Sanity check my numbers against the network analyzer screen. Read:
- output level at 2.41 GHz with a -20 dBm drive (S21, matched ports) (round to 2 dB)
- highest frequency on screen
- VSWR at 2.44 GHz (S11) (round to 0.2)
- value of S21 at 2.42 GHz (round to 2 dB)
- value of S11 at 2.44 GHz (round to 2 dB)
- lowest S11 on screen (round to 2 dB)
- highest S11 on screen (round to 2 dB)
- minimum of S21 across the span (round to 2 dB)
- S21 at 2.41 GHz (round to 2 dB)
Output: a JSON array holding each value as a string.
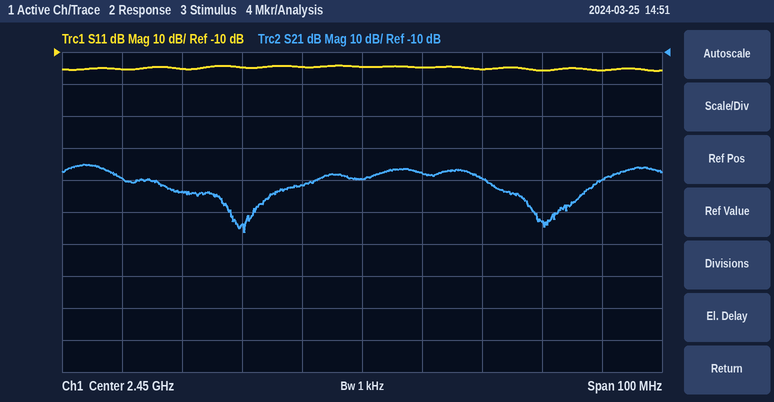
["-70 dBm", "2.5 GHz", "1.4", "-54 dB", "-14 dB", "-16 dB", "-14 dB", "-66 dB", "-50 dB"]
